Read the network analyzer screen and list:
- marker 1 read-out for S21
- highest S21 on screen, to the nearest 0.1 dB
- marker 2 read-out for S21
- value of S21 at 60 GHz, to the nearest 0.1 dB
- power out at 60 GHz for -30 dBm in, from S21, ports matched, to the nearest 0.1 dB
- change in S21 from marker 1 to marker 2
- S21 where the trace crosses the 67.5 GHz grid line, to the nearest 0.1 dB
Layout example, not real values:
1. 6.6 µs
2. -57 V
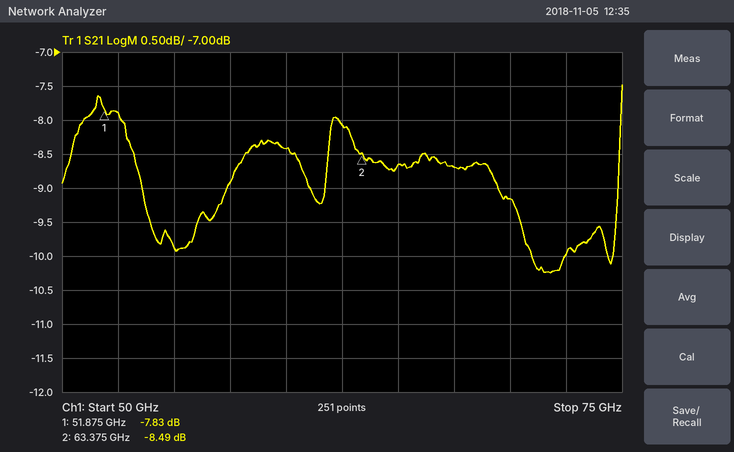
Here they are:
1. -7.83 dB
2. -7.5 dB
3. -8.49 dB
4. -8.4 dB
5. -38.4 dBm
6. -0.66 dB
7. -8.7 dB
